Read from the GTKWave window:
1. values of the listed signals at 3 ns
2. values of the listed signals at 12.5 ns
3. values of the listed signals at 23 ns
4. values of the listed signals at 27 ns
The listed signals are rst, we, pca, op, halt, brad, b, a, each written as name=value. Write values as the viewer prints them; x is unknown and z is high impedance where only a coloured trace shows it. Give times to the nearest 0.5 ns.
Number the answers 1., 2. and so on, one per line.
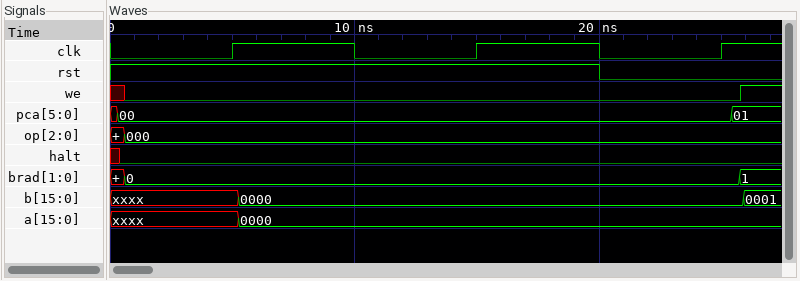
1. rst=1, we=0, pca=00, op=000, halt=0, brad=0, b=xxxx, a=xxxx
2. rst=1, we=0, pca=00, op=000, halt=0, brad=0, b=0000, a=0000
3. rst=0, we=0, pca=00, op=000, halt=0, brad=0, b=0000, a=0000
4. rst=0, we=1, pca=01, op=000, halt=0, brad=1, b=0001, a=0000
